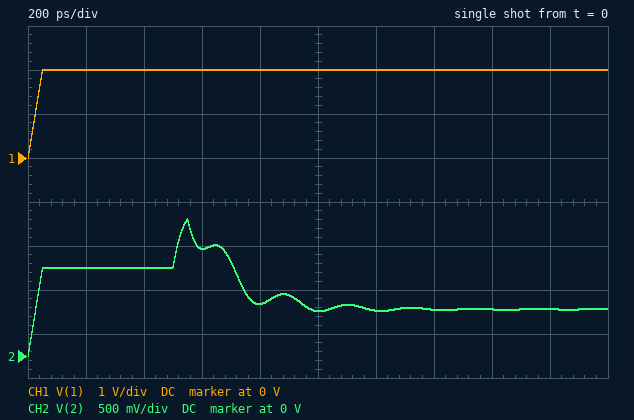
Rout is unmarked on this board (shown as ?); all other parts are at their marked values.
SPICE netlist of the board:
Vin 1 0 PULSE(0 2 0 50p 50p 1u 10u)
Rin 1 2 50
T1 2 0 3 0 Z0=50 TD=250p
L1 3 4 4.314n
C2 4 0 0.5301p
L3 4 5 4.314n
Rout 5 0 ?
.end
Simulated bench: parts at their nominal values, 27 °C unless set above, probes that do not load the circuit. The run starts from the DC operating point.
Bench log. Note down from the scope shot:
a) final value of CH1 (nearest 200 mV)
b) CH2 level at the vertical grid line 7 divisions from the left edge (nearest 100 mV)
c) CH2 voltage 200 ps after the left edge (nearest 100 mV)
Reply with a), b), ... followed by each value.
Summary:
a) 2.0 V
b) 500 mV
c) 1.0 V
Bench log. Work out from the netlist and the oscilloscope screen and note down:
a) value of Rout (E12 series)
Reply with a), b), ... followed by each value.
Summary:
a) 18 Ω
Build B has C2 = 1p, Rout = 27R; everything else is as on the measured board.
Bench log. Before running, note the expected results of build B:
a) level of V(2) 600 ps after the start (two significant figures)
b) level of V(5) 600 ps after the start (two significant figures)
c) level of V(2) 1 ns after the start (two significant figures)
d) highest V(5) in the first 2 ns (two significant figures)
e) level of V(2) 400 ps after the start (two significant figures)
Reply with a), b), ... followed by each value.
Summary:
a) 1.1 V
b) 630 mV
c) 760 mV
d) 720 mV
e) 1.0 V
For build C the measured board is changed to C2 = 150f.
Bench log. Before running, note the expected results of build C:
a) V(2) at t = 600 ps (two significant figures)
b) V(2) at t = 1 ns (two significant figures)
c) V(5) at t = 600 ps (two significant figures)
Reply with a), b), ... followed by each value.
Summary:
a) 1.5 V
b) 540 mV
c) 500 mV
